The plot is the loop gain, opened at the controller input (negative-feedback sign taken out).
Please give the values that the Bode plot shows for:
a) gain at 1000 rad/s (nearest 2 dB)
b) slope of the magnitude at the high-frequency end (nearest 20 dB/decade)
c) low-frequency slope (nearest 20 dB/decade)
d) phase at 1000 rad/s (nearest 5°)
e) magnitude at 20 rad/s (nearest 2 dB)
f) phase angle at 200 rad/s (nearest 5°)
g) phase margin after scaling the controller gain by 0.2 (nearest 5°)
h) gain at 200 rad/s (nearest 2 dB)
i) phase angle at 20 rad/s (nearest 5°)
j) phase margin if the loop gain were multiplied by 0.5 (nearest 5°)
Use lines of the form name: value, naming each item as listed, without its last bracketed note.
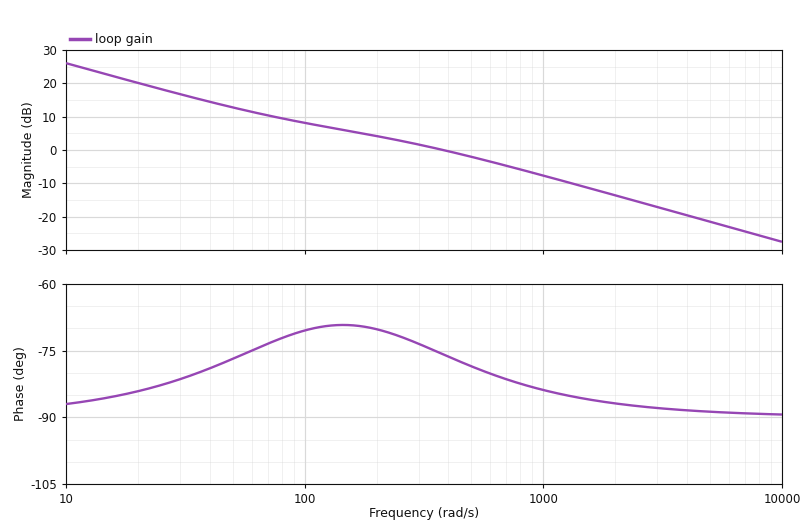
gain at 1000 rad/s: -8 dB
slope of the magnitude at the high-frequency end: -20 dB/decade
low-frequency slope: -20 dB/decade
phase at 1000 rad/s: -85°
magnitude at 20 rad/s: 20 dB
phase angle at 200 rad/s: -70°
phase margin after scaling the controller gain by 0.2: 100°
gain at 200 rad/s: 4 dB
phase angle at 20 rad/s: -85°
phase margin if the loop gain were multiplied by 0.5: 110°
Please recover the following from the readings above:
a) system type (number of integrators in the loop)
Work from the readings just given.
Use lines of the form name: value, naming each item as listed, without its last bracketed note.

system type: 1
